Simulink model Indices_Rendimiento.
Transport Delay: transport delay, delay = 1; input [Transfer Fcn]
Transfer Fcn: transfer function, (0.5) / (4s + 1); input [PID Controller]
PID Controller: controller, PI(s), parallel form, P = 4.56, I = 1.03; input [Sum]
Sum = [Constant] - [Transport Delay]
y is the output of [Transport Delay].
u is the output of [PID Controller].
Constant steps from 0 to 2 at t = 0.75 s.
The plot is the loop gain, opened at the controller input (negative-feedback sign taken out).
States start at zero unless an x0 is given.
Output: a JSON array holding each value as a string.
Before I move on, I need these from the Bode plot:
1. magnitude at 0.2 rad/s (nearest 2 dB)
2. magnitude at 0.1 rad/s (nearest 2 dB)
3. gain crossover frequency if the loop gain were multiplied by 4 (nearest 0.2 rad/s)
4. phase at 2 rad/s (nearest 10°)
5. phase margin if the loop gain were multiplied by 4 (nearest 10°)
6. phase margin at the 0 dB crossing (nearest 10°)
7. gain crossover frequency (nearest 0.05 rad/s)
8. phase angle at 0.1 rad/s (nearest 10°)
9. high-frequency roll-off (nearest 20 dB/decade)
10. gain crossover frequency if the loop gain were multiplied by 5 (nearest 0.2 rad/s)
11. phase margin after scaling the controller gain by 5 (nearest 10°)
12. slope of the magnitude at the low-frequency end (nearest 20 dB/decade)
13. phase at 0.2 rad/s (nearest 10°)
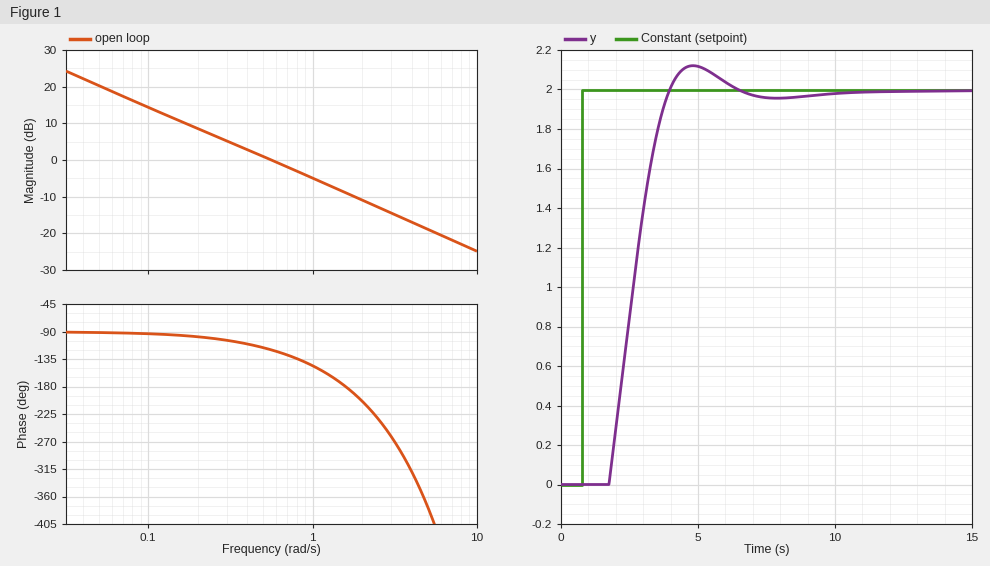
["8 dB", "14 dB", "2.2 rad/s", "-200°", "-40°", "60°", "0.55 rad/s", "-90°", "-20 dB/decade", "2.8 rad/s", "-70°", "-20 dB/decade", "-100°"]
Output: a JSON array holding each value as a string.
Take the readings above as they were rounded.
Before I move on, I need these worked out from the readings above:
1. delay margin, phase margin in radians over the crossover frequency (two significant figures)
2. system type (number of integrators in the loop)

["1.9 s", "1"]
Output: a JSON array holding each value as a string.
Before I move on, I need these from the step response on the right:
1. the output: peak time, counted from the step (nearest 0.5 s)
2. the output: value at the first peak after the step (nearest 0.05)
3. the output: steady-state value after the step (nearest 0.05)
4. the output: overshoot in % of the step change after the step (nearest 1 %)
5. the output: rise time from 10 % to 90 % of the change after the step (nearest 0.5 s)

["4.0 s", "2.10", "2.00", "6 %", "1.5 s"]
